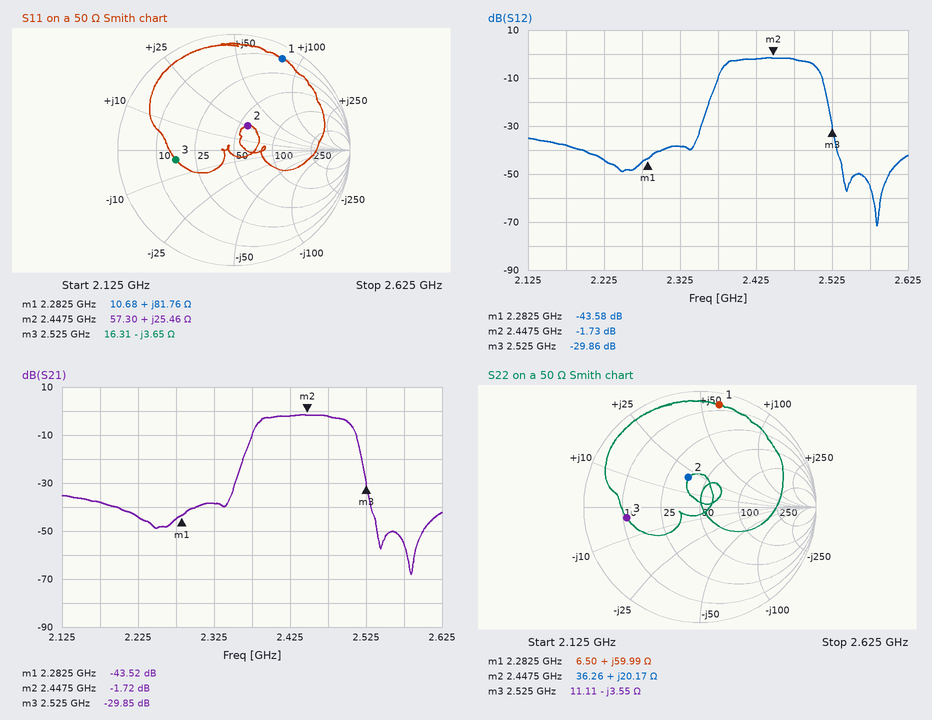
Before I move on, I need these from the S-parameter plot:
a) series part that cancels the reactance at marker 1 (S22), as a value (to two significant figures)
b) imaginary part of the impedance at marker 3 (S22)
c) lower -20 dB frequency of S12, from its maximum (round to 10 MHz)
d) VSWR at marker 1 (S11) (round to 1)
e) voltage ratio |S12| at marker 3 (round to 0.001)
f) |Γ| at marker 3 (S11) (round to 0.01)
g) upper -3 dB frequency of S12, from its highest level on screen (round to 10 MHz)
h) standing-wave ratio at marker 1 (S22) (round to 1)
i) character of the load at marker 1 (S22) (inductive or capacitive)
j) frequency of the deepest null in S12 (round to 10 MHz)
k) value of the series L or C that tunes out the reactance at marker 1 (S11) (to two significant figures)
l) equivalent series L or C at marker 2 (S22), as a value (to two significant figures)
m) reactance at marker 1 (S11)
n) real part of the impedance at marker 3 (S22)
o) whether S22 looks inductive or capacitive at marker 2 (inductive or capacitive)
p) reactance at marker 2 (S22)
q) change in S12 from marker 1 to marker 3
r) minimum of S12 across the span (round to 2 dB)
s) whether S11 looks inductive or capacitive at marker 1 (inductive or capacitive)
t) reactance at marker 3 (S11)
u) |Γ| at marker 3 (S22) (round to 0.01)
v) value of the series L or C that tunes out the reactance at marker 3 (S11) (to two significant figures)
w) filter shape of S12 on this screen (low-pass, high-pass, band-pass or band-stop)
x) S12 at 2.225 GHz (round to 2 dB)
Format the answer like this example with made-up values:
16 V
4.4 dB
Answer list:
1.2 pF
-3.55 Ω
2.36 GHz
17
0.032
0.51
2.50 GHz
19
inductive
2.58 GHz
850 fF
1.3 nH
+81.76 Ω
11.11 Ω
inductive
+20.17 Ω
13.72 dB
-72 dB
inductive
-3.65 Ω
0.64
230 pH
band-pass
-44 dB
